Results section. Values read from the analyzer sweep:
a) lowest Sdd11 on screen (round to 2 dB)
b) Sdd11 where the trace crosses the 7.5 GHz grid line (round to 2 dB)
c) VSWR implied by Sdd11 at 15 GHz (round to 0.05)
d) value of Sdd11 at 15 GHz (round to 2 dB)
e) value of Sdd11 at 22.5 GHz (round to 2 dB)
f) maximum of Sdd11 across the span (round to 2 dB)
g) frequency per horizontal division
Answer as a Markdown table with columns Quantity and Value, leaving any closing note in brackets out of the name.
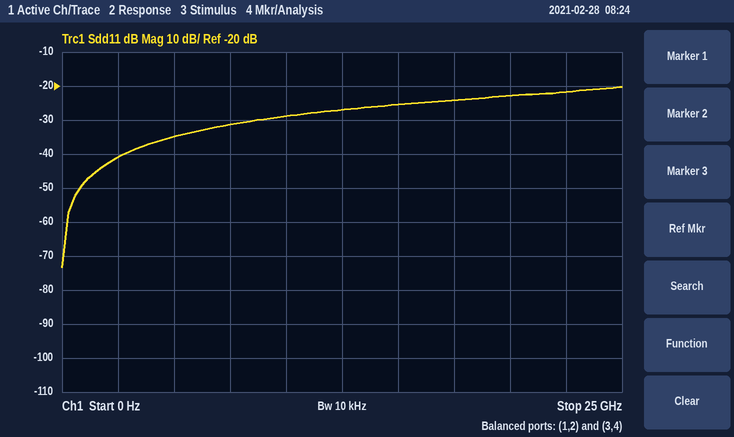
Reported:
| Quantity | Value |
|---|---|
| lowest Sdd11 on screen | -74 dB |
| Sdd11 where the trace crosses the 7.5 GHz grid line | -32 dB |
| VSWR implied by Sdd11 at 15 GHz | 1.10 |
| value of Sdd11 at 15 GHz | -26 dB |
| value of Sdd11 at 22.5 GHz | -22 dB |
| maximum of Sdd11 across the span | -20 dB |
| frequency per horizontal division | 2.5 GHz |
